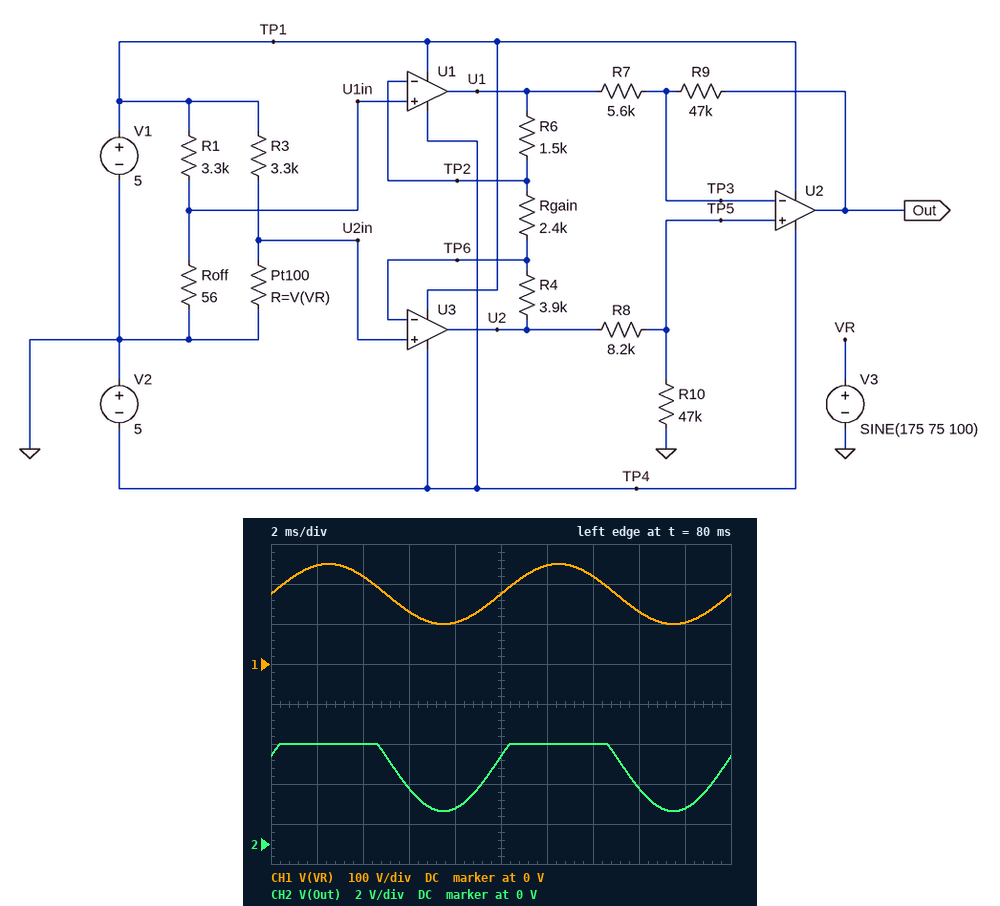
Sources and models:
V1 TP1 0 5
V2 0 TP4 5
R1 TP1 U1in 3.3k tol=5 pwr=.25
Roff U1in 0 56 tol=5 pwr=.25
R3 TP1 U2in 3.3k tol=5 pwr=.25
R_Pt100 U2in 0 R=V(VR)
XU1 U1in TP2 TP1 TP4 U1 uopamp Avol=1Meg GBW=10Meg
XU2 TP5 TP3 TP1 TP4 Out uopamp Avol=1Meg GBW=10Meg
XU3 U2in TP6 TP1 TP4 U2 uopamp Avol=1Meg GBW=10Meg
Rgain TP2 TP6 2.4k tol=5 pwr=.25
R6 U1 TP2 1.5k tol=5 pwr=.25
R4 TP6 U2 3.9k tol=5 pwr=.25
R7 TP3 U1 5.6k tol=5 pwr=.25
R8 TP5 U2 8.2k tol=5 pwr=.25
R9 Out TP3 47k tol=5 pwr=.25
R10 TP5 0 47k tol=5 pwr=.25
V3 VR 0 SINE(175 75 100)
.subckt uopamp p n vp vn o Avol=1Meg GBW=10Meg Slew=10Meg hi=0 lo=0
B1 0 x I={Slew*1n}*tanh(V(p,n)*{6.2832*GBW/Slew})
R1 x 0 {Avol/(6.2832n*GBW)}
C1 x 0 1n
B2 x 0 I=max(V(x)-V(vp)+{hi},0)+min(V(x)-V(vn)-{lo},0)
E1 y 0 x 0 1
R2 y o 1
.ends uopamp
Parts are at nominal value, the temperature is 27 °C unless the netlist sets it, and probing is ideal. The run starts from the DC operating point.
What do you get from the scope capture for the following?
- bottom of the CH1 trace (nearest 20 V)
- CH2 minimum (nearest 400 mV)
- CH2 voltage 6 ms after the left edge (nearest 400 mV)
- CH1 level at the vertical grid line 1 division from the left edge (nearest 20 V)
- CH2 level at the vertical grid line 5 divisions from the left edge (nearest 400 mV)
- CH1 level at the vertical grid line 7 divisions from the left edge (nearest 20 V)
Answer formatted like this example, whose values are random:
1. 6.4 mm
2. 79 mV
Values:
1. 100 V
2. 1.6 V
3. 2.8 V
4. 240 V
5. 4.4 V
6. 220 V
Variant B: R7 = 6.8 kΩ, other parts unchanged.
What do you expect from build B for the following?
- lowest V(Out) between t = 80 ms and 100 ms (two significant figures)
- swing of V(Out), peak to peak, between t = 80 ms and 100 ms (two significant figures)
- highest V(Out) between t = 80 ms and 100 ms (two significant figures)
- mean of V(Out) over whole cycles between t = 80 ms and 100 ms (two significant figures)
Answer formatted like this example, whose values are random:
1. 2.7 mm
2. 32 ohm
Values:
1. 1.4 V
2. 3.6 V
3. 5.0 V
4. 3.5 V
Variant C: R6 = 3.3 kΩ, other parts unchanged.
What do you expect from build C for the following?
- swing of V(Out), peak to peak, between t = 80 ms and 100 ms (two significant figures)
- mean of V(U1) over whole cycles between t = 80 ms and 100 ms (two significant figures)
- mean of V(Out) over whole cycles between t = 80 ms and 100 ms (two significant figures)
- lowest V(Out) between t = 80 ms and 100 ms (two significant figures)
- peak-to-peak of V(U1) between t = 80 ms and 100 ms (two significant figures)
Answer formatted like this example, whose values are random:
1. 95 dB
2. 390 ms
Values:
1. 3.0 V
2. -150 mV
3. 4.1 V
4. 2.0 V
5. 280 mV
